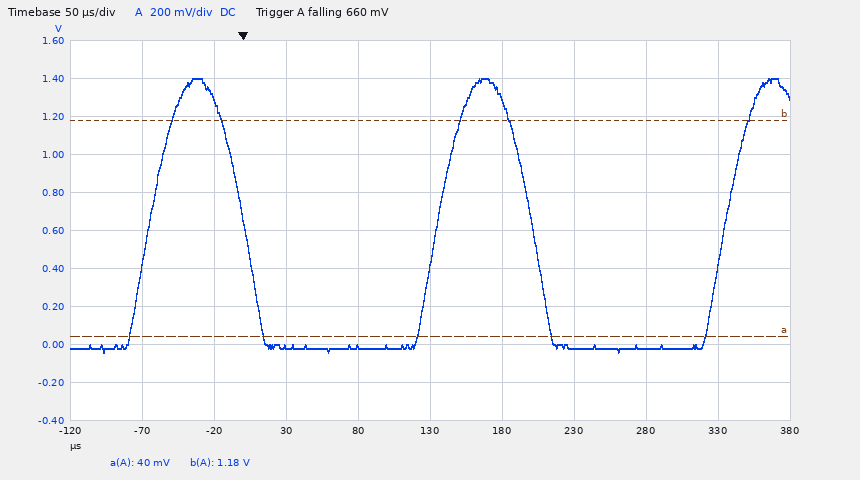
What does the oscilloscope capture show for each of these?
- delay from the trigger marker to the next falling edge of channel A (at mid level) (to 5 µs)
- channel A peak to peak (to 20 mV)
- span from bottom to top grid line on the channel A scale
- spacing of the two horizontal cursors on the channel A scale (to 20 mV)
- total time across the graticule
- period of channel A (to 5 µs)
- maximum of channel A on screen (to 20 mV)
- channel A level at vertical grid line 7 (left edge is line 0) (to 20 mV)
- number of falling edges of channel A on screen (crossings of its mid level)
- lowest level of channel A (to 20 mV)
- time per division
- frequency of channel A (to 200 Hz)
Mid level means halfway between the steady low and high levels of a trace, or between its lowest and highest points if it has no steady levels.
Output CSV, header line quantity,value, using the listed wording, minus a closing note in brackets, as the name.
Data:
quantity,value
delay from the trigger marker to the next falling edge of channel A (at mid level),200 µs
channel A peak to peak,1.44 V
span from bottom to top grid line on the channel A scale,2 V
spacing of the two horizontal cursors on the channel A scale,1.14 V
total time across the graticule,500 µs
period of channel A,200 µs
maximum of channel A on screen,1.40 V
channel A level at vertical grid line 7 (left edge is line 0),-20 mV
number of falling edges of channel A on screen,2
lowest level of channel A,-40 mV
time per division,50 µs
frequency of channel A,5.0 kHz
